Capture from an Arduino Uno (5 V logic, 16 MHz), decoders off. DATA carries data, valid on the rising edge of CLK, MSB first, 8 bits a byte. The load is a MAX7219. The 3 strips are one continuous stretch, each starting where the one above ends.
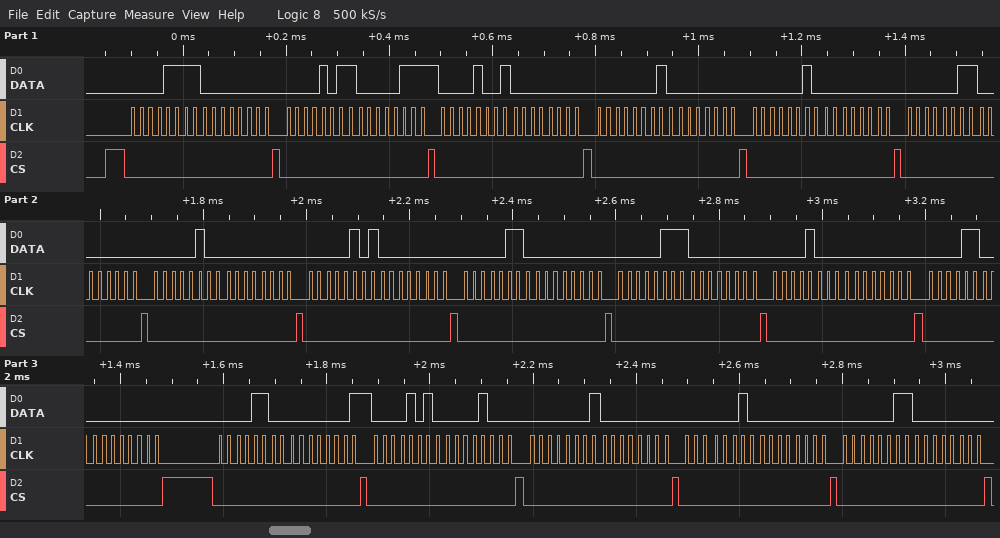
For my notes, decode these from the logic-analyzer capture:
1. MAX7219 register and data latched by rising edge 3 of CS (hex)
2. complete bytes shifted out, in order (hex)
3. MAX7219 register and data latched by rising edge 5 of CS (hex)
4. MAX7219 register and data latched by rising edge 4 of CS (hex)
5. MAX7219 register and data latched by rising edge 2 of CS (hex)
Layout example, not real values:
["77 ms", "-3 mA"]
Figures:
["register 0xB, data 0x07", "0F 00 0B 07 09 00 01 00 02 00 03 00 04 00 05 00 06 00 07 00 08 00 0C 00 0C 01 0A 08 01 00 02 00 03 00", "register 0x1, data 0x00", "register 0x9, data 0x00", "register 0xF, data 0x00"]
